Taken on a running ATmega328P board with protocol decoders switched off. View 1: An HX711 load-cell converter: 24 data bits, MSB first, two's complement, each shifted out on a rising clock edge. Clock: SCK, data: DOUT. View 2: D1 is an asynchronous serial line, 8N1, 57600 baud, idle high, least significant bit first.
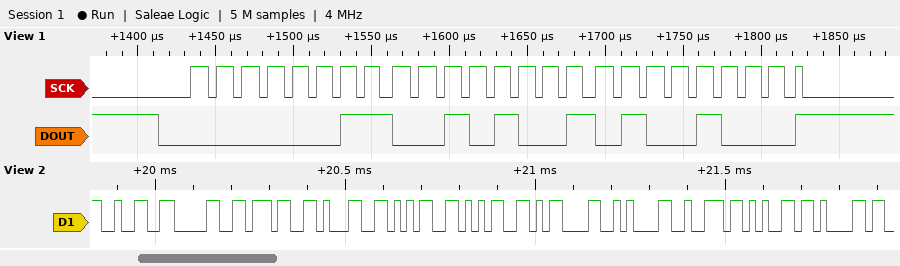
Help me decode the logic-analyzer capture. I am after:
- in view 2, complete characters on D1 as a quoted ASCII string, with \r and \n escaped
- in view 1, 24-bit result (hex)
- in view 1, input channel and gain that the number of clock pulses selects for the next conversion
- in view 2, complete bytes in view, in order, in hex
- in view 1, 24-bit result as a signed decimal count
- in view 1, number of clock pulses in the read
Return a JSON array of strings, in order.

["\"207155\\r\\nrea\"", "0x032948", "channel A, gain 128", "32 30 37 31 35 35 0D 0A 72 65 61", "207176", "25"]
